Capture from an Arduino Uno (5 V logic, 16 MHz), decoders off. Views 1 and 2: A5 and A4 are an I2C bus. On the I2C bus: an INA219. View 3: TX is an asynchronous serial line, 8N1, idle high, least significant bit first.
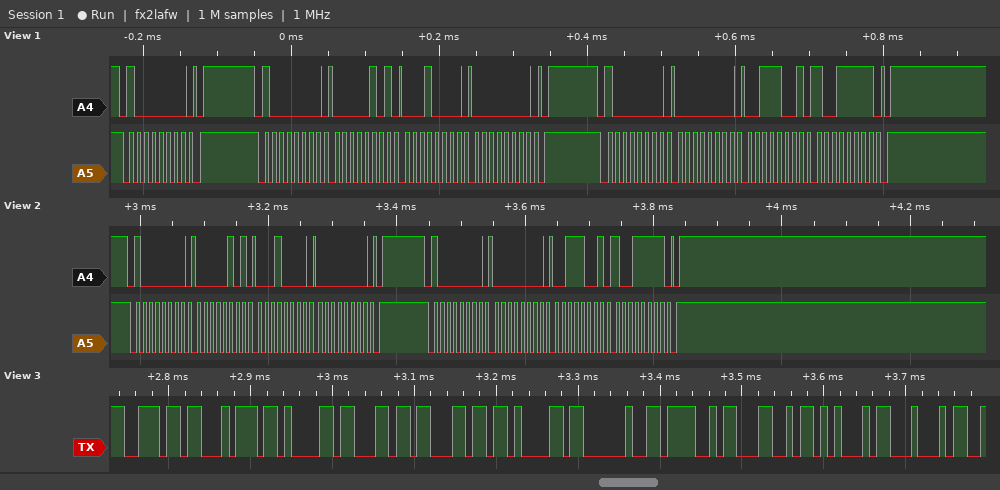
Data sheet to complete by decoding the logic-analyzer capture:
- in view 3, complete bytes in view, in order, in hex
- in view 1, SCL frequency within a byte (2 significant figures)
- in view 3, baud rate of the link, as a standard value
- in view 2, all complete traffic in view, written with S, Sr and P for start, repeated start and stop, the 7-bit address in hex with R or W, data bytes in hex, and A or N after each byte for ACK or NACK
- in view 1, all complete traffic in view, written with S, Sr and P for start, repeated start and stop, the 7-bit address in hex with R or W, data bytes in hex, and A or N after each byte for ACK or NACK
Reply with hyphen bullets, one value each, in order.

- 6E 74 61 6C 6C 61 20 4F 4C 45 44
- 100 kHz
- 115200 baud
- S 40W A 05 A 10 A 00 A P S 40W A 00 A 39 A 9F A P
- S 40W A P S 40W A 05 A 10 A 00 A P S 40W A 00 A 39 A 9F A P
